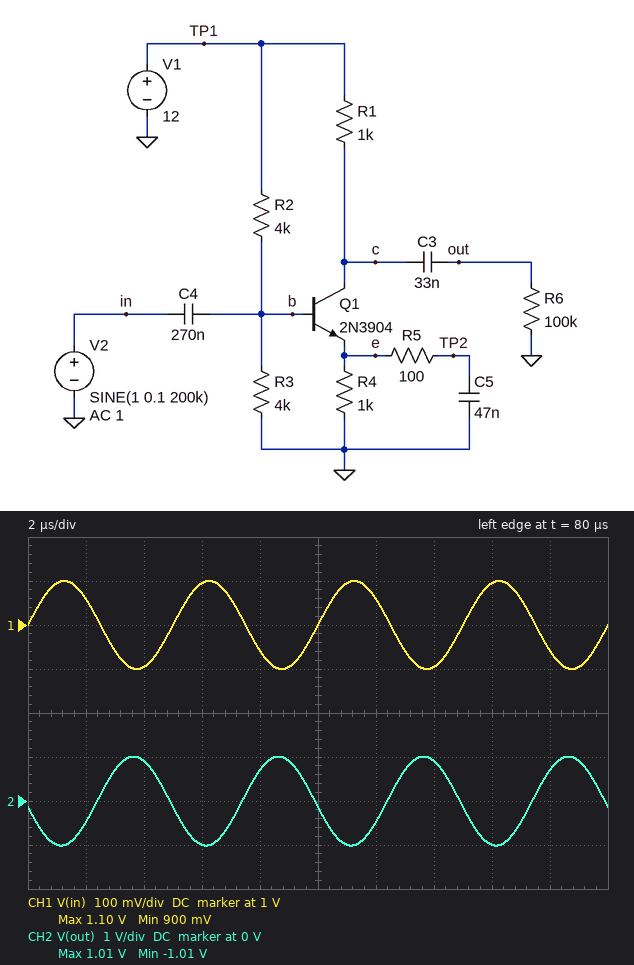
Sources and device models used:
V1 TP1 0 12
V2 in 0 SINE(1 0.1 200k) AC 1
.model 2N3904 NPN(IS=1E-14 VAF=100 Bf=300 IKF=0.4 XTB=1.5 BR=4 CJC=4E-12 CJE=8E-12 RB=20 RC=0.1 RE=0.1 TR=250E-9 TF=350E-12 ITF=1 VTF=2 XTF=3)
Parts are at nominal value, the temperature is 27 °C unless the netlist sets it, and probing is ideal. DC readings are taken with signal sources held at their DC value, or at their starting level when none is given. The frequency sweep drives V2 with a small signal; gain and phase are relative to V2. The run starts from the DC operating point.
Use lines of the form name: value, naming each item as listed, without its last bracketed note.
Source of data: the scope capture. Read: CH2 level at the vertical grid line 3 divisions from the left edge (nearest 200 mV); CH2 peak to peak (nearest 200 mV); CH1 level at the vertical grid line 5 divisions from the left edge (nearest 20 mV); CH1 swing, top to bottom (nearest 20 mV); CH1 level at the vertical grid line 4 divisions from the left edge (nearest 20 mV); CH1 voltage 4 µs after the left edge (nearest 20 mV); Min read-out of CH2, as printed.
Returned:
CH2 level at the vertical grid line 3 divisions from the left edge: -1.0 V
CH2 peak to peak: 2.0 V
CH1 level at the vertical grid line 5 divisions from the left edge: 1.00 V
CH1 swing, top to bottom: 200 mV
CH1 level at the vertical grid line 4 divisions from the left edge: 940 mV
CH1 voltage 4 µs after the left edge: 900 mV
Min read-out of CH2, as printed: -1.01 V
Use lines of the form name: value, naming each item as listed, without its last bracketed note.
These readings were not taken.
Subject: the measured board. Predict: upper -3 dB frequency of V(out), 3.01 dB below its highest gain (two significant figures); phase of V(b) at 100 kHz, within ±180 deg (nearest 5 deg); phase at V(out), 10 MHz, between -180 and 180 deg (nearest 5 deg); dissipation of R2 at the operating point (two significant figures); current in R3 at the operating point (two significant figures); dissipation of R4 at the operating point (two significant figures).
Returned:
upper -3 dB frequency of V(out), 3.01 dB below its highest gain: 41 MHz
phase of V(b) at 100 kHz, within ±180 deg: 0 deg
phase at V(out), 10 MHz, between -180 and 180 deg: 165 deg
dissipation of R2 at the operating point: 9.1 mW
current in R3 at the operating point: 1.5 mA
dissipation of R4 at the operating point: 28 mW
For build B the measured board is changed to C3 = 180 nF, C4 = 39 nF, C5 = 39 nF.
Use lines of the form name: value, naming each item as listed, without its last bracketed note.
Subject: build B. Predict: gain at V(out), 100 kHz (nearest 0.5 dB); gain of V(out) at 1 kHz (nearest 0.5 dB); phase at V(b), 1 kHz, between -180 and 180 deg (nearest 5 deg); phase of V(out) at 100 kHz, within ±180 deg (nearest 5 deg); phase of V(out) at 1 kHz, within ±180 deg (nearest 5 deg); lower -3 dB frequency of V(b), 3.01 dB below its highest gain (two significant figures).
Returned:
gain at V(out), 100 kHz: 19.5 dB
gain of V(out) at 1 kHz: -7.0 dB
phase at V(b), 1 kHz, between -180 and 180 deg: 65 deg
phase of V(out) at 100 kHz, within ±180 deg: -160 deg
phase of V(out) at 1 kHz, within ±180 deg: -100 deg
lower -3 dB frequency of V(b), 3.01 dB below its highest gain: 2.1 kHz
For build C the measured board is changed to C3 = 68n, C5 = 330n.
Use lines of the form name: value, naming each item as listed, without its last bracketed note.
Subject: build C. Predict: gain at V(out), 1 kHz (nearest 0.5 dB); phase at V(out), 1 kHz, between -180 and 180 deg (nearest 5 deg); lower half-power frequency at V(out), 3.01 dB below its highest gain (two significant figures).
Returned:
gain at V(out), 1 kHz: 7.0 dB
phase at V(out), 1 kHz, between -180 and 180 deg: -110 deg
lower half-power frequency at V(out), 3.01 dB below its highest gain: 4.6 kHz
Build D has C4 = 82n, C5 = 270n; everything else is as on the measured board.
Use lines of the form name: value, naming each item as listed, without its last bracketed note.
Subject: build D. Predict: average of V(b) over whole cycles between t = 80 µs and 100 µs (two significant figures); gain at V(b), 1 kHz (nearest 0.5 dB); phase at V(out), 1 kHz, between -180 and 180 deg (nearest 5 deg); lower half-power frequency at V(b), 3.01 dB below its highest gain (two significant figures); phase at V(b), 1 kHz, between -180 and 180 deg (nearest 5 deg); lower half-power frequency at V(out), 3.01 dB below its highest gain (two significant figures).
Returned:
average of V(b) over whole cycles between t = 80 µs and 100 µs: 6.0 V
gain at V(b), 1 kHz: -3.0 dB
phase at V(out), 1 kHz, between -180 and 180 deg: -80 deg
lower half-power frequency at V(b), 3.01 dB below its highest gain: 990 Hz
phase at V(b), 1 kHz, between -180 and 180 deg: 45 deg
lower half-power frequency at V(out), 3.01 dB below its highest gain: 5.8 kHz
